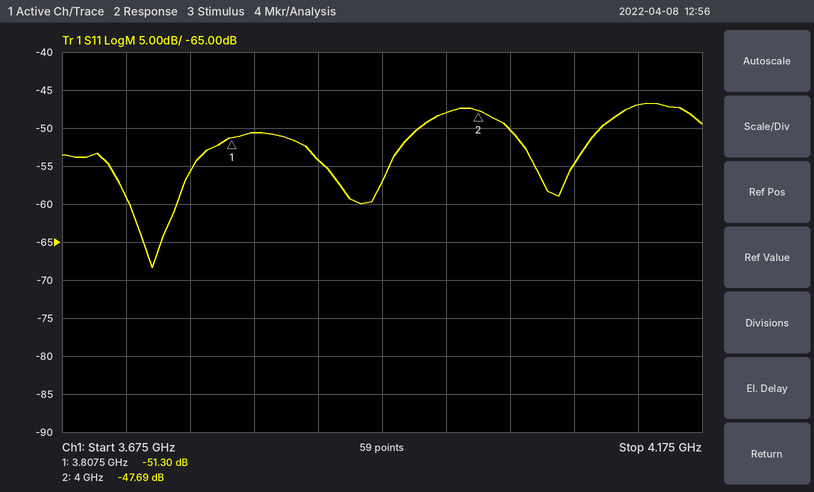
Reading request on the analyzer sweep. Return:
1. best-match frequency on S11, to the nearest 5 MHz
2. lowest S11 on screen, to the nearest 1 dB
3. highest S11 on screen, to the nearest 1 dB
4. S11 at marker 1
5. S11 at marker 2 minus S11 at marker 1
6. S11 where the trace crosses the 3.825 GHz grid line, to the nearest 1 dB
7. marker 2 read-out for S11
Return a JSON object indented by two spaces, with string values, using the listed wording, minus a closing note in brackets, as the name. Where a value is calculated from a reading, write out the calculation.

{
  "best-match frequency on S11, to the nearest 5 MHz": "3.745 GHz",
  "lowest S11 on screen, to the nearest 1 dB": "-68 dB",
  "highest S11 on screen, to the nearest 1 dB": "-47 dB",
  "S11 at marker 1": "-51.30 dB",
  "S11 at marker 2 minus S11 at marker 1": "-47.69 − (-51.3) = 3.61 dB",
  "S11 where the trace crosses the 3.825 GHz grid line, to the nearest 1 dB": "-51 dB",
  "marker 2 read-out for S11": "-47.69 dB"
}
